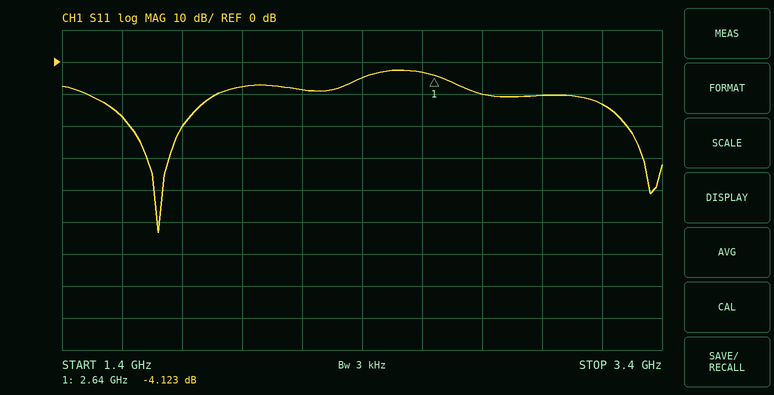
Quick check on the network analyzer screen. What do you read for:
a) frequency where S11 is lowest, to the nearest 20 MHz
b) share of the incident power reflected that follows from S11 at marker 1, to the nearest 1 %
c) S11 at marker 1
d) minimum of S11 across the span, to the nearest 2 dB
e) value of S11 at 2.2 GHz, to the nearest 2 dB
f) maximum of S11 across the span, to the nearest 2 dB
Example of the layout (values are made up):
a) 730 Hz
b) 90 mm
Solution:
a) 1.72 GHz
b) 39 %
c) -4.123 dB
d) -54 dB
e) -8 dB
f) -2 dB
